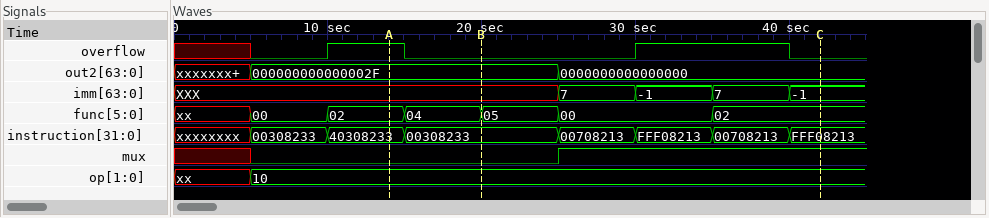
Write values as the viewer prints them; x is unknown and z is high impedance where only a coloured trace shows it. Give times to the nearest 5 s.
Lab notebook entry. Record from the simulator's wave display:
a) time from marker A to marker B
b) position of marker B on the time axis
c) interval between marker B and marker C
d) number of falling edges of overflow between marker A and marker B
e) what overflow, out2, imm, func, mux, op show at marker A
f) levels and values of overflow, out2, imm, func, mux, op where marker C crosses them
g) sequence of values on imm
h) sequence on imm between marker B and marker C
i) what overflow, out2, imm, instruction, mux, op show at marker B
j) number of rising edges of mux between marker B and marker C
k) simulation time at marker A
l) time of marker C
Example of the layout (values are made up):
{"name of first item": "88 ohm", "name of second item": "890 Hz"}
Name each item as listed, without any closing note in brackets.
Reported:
{"time from marker A to marker B": "5 s", "position of marker B on the time axis": "20 s", "interval between marker B and marker C": "20 s", "number of falling edges of overflow between marker A and marker B": "1", "what overflow, out2, imm, func, mux, op show at marker A": "overflow=1, out2=000000000000002F, imm=XXX, func=02, mux=0, op=10", "levels and values of overflow, out2, imm, func, mux, op where marker C crosses them": "overflow=0, out2=0000000000000000, imm=-1, func=02, mux=1, op=10", "sequence of values on imm": "XXX, 7, -1, 7, -1", "sequence on imm between marker B and marker C": "XXX, 7, -1, 7, -1", "what overflow, out2, imm, instruction, mux, op show at marker B": "overflow=0, out2=000000000000002F, imm=XXX, instruction=00308233, mux=0, op=10", "number of rising edges of mux between marker B and marker C": "1", "simulation time at marker A": "15 s", "time of marker C": "40 s"}
